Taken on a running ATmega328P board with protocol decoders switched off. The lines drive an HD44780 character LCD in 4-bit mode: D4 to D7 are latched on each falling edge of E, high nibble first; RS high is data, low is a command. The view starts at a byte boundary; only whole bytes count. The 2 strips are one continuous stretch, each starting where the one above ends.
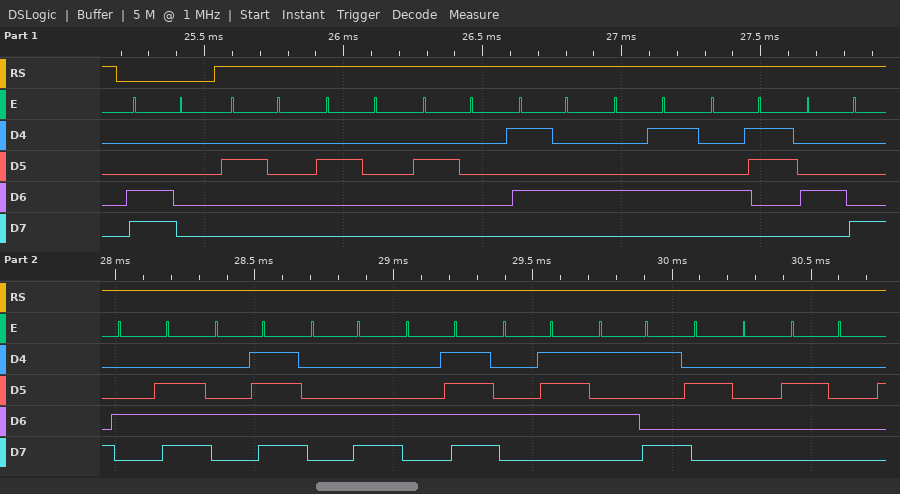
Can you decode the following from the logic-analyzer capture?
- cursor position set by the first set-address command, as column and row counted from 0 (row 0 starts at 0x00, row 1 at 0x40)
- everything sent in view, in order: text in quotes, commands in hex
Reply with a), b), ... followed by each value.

a) column 0, row 1
b) 0xC0 "   TECHNOLOGY  "
